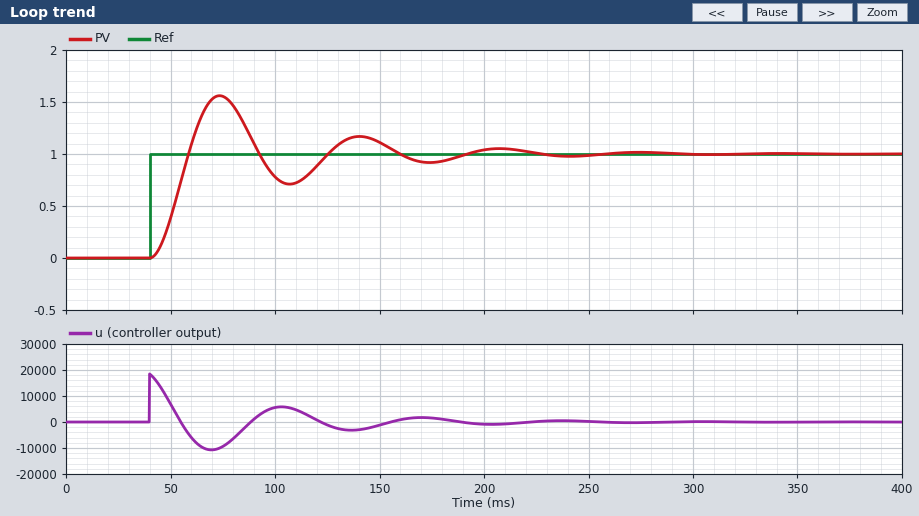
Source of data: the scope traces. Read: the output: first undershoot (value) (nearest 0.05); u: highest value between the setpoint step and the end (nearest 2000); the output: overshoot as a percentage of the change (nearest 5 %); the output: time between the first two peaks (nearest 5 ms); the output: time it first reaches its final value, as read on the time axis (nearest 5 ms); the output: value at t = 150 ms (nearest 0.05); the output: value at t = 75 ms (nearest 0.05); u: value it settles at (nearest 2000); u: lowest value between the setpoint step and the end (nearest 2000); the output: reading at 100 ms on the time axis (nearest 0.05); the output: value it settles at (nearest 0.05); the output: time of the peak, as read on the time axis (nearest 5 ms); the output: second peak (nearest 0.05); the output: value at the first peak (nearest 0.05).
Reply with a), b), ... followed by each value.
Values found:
a) 0.70
b) 18000
c) 55 %
d) 65 ms
e) 60 ms
f) 1.10
g) 1.55
h) 0
i) -10000
j) 0.80
k) 1.00
l) 75 ms
m) 1.15
n) 1.55
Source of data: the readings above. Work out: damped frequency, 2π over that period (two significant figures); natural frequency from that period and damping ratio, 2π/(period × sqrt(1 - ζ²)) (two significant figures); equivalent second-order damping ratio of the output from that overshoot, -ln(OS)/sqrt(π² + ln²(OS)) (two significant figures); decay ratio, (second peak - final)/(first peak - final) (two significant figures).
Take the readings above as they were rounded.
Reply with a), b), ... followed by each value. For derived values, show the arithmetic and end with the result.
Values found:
a) 2π / 65 = 0.097 rad/ms
b) 2π / (65 × sqrt(1 - 0.19²)) = 0.098 rad/ms
c) ln(0.55) = -0.598; 0.598 / sqrt(9.870 + 0.357) = 0.19
d) (1.15 - 1) / (1.55 - 1) = 0.27
